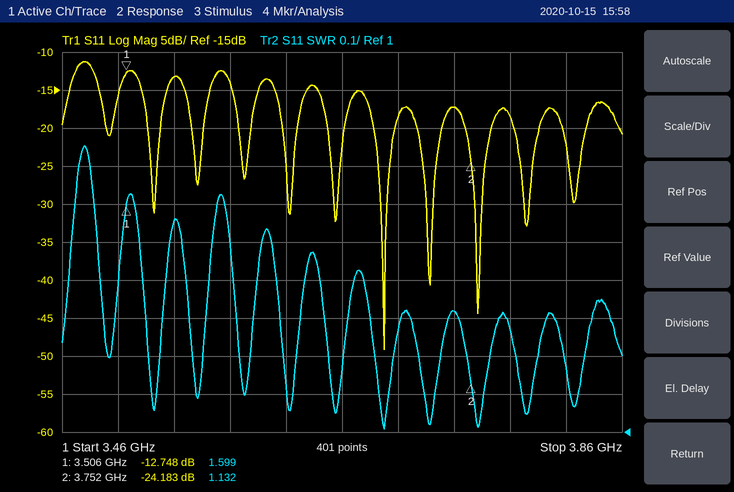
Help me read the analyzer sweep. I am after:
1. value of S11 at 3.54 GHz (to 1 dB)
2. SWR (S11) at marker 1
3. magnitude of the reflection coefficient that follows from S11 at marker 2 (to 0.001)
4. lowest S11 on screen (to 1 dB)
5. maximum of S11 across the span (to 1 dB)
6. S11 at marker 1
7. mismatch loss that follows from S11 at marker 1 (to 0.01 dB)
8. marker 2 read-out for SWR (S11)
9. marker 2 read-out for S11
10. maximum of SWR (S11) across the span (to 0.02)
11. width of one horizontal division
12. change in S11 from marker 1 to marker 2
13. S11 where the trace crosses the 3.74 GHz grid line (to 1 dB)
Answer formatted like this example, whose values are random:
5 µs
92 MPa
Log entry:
-13 dB
1.599
0.062
-49 dB
-11 dB
-12.748 dB
0.24 dB
1.132
-24.183 dB
1.76
40 MHz
-11.435 dB
-17 dB
